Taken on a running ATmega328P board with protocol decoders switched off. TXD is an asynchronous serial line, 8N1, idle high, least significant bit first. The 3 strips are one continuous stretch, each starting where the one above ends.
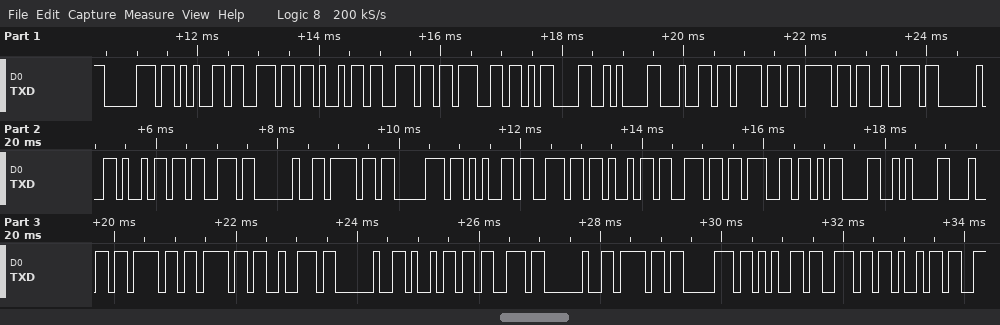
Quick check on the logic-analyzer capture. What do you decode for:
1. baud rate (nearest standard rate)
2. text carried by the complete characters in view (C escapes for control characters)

9600 baud
"pening\r\ndoor is opening\r\ndoor is openi"
